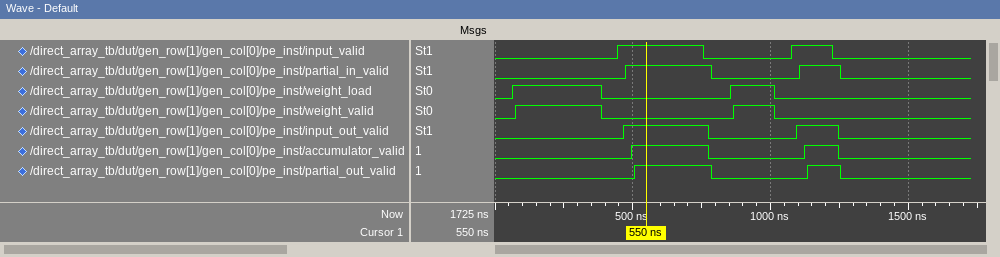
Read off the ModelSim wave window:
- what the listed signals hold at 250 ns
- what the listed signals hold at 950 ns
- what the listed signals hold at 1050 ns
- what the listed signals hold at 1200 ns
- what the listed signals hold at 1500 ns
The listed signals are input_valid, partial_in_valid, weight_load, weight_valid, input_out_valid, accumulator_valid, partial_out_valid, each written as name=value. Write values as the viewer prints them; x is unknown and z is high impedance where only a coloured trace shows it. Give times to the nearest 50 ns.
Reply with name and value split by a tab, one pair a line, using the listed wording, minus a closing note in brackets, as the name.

what the listed signals hold at 250 ns	input_valid=0, partial_in_valid=0, weight_load=1, weight_valid=1, input_out_valid=0, accumulator_valid=0, partial_out_valid=0
what the listed signals hold at 950 ns	input_valid=0, partial_in_valid=0, weight_load=1, weight_valid=1, input_out_valid=0, accumulator_valid=0, partial_out_valid=0
what the listed signals hold at 1050 ns	input_valid=0, partial_in_valid=0, weight_load=0, weight_valid=0, input_out_valid=0, accumulator_valid=0, partial_out_valid=0
what the listed signals hold at 1200 ns	input_valid=1, partial_in_valid=1, weight_load=0, weight_valid=0, input_out_valid=1, accumulator_valid=1, partial_out_valid=1
what the listed signals hold at 1500 ns	input_valid=0, partial_in_valid=0, weight_load=0, weight_valid=0, input_out_valid=0, accumulator_valid=0, partial_out_valid=0
